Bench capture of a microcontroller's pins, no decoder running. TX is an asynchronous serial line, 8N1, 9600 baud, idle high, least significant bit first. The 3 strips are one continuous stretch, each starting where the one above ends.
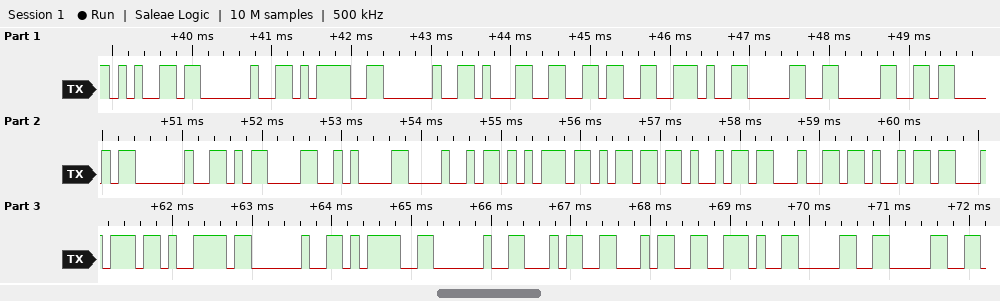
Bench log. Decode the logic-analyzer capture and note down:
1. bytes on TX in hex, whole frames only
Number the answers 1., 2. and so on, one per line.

1. 0x65 0x20 0x3D 0x20 0x31 0x36 0x2E 0x30 0x30 0x43 0x20 0x0D 0x0A 0x48 0x75 0x6D 0x69 0x64 0x69 0x74 0x79 0x20 0x3D 0x20 0x34 0x34 0x2E 0x30 0x30
